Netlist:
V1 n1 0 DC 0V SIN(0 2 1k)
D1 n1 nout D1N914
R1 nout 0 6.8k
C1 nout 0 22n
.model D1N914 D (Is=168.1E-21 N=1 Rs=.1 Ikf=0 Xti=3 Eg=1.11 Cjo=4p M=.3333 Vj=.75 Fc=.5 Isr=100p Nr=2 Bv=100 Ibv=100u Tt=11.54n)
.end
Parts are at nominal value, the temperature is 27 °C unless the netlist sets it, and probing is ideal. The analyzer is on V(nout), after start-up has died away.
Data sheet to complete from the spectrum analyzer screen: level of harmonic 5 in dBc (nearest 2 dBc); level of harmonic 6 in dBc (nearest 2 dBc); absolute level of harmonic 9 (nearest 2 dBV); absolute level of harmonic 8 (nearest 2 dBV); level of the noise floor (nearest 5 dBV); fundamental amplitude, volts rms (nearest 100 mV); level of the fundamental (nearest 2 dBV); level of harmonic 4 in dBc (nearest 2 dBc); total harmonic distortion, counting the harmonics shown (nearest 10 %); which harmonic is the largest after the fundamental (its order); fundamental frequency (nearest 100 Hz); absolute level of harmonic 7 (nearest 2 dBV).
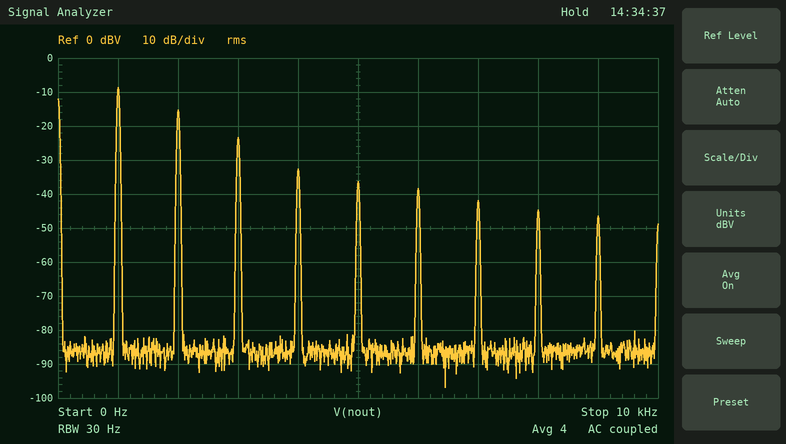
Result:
-28 dBc
-30 dBc
-46 dBV
-44 dBV
-85 dBV
400 mV
-8 dBV
-24 dBc
50 %
2
1.0 kHz
-42 dBV
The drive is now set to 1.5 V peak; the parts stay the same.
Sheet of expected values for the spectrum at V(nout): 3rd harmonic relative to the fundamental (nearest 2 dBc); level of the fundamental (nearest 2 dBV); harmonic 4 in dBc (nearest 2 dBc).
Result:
-14 dBc
-14 dBV
-22 dBc
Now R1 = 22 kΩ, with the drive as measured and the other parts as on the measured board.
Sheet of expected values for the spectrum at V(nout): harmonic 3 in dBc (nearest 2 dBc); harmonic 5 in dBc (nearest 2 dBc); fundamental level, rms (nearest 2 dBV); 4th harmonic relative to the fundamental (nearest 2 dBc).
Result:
-14 dBc
-26 dBc
-10 dBV
-20 dBc
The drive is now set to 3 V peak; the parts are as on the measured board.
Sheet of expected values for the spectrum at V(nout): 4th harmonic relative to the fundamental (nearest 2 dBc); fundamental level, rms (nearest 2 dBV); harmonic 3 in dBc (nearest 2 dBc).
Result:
-26 dBc
-4 dBV
-16 dBc
